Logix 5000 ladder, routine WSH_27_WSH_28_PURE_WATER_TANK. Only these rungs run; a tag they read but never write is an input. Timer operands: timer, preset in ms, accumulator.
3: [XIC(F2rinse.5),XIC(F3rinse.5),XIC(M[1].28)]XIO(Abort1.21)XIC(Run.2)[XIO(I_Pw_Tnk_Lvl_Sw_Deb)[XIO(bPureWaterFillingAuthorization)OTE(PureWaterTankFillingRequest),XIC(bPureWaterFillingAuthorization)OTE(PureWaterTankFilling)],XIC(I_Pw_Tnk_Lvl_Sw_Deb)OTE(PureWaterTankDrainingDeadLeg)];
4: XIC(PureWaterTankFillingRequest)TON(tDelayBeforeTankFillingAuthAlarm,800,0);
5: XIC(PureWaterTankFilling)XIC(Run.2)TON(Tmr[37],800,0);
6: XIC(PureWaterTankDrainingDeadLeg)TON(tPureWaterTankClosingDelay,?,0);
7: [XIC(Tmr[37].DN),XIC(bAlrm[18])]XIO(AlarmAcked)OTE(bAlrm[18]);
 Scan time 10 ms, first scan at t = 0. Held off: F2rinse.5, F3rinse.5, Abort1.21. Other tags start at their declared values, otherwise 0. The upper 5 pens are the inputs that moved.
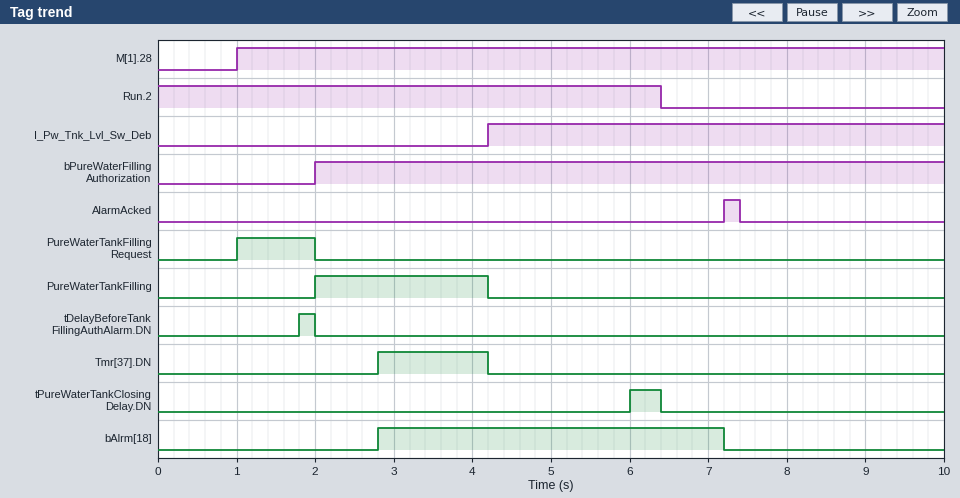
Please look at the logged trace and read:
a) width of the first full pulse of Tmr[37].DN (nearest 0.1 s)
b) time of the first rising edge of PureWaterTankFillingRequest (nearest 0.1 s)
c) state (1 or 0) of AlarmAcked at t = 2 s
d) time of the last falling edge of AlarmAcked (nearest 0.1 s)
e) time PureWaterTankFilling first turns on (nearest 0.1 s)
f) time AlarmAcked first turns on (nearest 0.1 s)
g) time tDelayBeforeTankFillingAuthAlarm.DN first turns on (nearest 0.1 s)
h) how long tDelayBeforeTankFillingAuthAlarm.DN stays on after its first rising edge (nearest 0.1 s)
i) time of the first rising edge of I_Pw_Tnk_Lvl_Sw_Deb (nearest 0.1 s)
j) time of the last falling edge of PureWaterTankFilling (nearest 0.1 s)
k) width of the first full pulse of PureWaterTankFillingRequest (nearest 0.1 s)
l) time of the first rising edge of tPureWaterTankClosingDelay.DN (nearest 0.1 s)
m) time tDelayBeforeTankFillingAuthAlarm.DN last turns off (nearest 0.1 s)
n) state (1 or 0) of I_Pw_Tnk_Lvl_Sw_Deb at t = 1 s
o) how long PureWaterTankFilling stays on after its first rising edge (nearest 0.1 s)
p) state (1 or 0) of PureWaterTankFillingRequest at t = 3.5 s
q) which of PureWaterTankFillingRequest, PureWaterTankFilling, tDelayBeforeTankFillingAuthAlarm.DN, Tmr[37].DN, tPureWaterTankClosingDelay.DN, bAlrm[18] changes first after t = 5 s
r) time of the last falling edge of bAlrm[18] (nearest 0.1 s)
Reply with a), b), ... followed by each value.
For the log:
a) 1.4 s
b) 1.0 s
c) 0
d) 7.4 s
e) 2.0 s
f) 7.2 s
g) 1.8 s
h) 0.2 s
i) 4.2 s
j) 4.2 s
k) 1.0 s
l) 6.0 s
m) 2.0 s
n) 0
o) 2.2 s
p) 0
q) tPureWaterTankClosingDelay.DN
r) 7.2 s
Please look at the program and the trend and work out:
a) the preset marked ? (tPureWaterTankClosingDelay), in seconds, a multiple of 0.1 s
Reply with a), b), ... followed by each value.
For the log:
a) 1.8 s
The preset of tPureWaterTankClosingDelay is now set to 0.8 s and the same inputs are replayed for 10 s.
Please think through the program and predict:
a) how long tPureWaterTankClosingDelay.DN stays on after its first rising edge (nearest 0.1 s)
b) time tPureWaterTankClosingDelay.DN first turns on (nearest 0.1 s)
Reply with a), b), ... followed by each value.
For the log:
a) 1.4 s
b) 5.0 s
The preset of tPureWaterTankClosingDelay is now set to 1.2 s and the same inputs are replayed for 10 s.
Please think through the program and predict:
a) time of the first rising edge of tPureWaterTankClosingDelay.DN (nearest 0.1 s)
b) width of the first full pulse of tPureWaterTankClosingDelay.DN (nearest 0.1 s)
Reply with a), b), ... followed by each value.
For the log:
a) 5.4 s
b) 1.0 s
